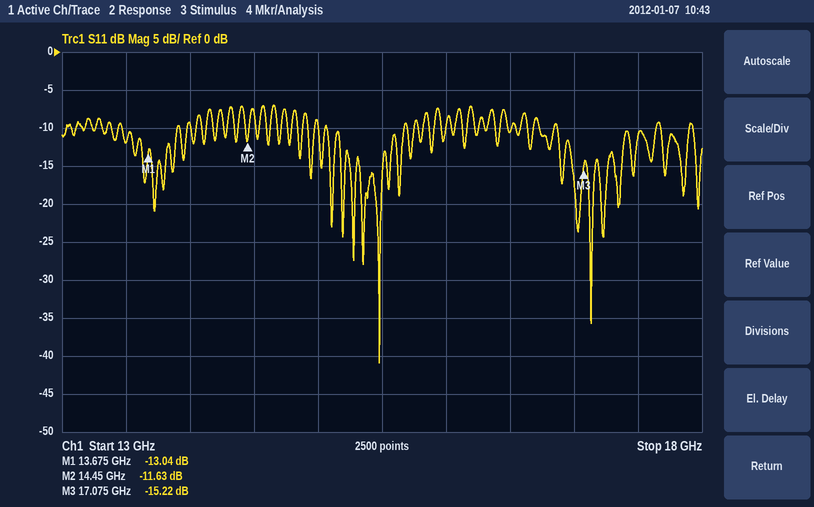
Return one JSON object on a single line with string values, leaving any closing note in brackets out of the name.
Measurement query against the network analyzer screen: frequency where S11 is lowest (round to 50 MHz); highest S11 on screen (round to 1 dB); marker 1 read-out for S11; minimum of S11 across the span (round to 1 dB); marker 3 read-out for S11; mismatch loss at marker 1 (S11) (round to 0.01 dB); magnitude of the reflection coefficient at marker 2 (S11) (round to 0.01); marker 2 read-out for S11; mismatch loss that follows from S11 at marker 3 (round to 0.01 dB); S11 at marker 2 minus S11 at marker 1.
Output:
{"frequency where S11 is lowest": "15.50 GHz", "highest S11 on screen": "-7 dB", "marker 1 read-out for S11": "-13.04 dB", "minimum of S11 across the span": "-41 dB", "marker 3 read-out for S11": "-15.22 dB", "mismatch loss at marker 1 (S11)": "0.22 dB", "magnitude of the reflection coefficient at marker 2 (S11)": "0.26", "marker 2 read-out for S11": "-11.63 dB", "mismatch loss that follows from S11 at marker 3": "0.13 dB", "S11 at marker 2 minus S11 at marker 1": "1.41 dB"}
